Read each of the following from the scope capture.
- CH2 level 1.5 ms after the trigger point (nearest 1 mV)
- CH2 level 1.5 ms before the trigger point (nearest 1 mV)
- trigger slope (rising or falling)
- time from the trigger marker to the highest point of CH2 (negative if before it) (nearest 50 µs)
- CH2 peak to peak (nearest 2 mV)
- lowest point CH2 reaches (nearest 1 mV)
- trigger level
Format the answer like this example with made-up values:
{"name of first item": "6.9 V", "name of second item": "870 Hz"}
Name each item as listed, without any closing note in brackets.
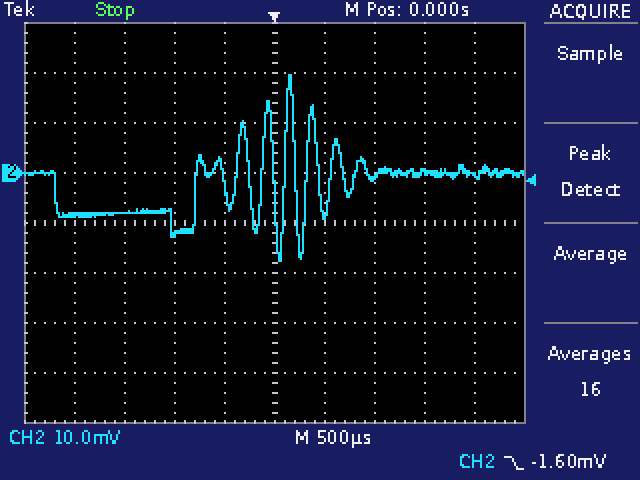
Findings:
{"CH2 level 1.5 ms after the trigger point": "0 mV", "CH2 level 1.5 ms before the trigger point": "-8 mV", "trigger slope": "falling", "time from the trigger marker to the highest point of CH2 (negative if before it)": "+150 µs", "CH2 peak to peak": "38 mV", "lowest point CH2 reaches": "-18 mV", "trigger level": "-1.60 mV"}
